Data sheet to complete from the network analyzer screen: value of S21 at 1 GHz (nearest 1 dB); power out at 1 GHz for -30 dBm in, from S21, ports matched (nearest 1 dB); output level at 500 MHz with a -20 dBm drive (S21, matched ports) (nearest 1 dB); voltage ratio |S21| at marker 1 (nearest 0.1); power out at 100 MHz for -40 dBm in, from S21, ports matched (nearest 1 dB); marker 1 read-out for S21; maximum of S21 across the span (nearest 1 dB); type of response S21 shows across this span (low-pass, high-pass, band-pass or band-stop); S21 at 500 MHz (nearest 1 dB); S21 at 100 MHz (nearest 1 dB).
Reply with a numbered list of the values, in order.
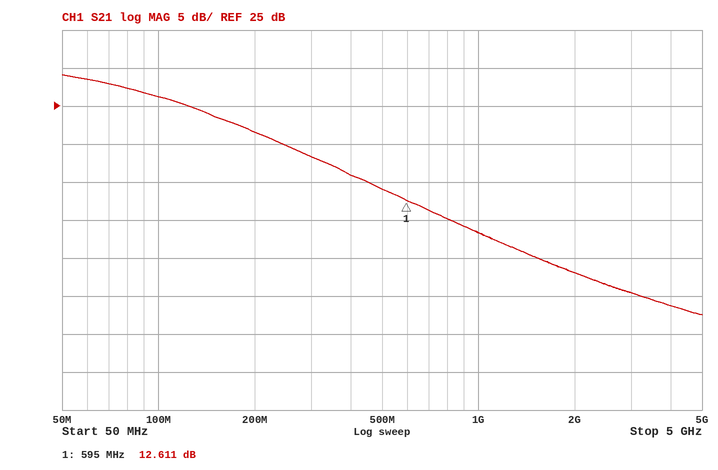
1. 8 dB
2. -22 dBm
3. -6 dBm
4. 4.3
5. -14 dBm
6. 12.611 dB
7. 29 dB
8. low-pass
9. 14 dB
10. 26 dB
